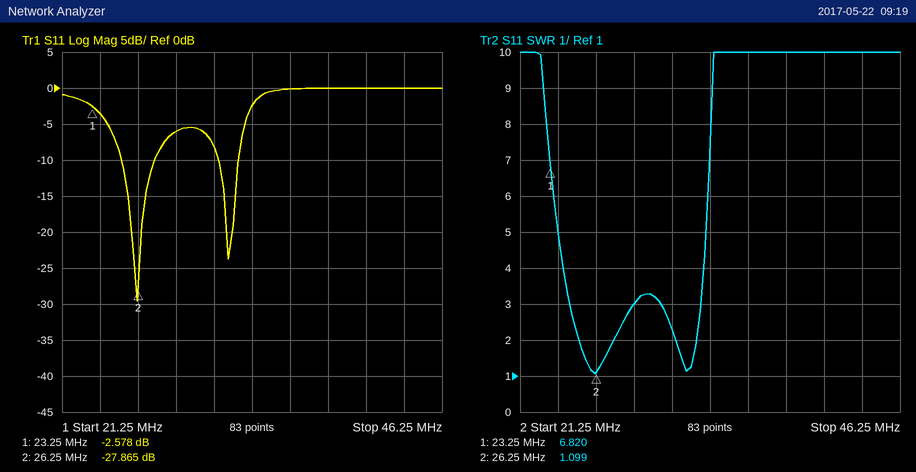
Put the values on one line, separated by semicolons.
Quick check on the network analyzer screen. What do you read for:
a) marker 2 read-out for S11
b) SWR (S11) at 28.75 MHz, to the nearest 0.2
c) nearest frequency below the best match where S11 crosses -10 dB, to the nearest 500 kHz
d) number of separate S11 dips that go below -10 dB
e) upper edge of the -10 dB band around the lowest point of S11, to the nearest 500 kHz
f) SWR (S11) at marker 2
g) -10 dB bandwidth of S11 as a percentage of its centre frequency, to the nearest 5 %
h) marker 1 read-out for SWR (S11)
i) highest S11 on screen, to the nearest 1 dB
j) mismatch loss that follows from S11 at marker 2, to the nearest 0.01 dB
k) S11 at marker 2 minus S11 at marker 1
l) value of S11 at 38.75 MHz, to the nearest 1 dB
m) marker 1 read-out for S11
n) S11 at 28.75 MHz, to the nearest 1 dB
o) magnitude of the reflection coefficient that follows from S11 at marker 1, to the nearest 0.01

-27.865 dB; 3.0; 25.0 MHz; 2; 27.5 MHz; 1.099; 10 %; 6.820; 0 dB; 0.01 dB; -25.287 dB; 0 dB; -2.578 dB; -6 dB; 0.74
